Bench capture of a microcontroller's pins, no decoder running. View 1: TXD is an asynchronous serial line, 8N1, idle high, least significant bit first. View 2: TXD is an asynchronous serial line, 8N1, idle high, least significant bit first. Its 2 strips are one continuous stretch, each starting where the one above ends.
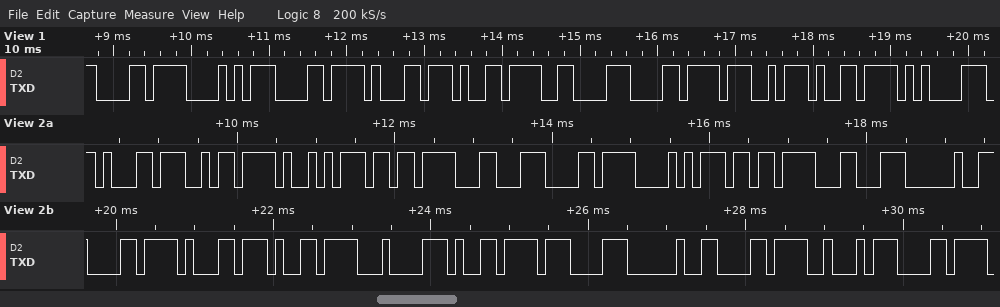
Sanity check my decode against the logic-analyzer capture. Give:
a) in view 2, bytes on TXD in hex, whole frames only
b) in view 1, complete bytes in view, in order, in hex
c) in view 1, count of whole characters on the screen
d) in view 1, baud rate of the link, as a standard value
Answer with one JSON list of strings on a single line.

["B1 DA A9 DB 8C D8 A8 DB 8C 20 D8 B1 D9 84 D9 87 20 D8 A2 D8", "D8 A8 D8 B1 D9 86 D8 A7 D9 85", "10", "9600 baud"]
